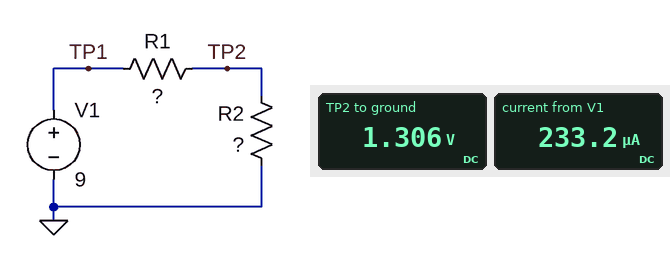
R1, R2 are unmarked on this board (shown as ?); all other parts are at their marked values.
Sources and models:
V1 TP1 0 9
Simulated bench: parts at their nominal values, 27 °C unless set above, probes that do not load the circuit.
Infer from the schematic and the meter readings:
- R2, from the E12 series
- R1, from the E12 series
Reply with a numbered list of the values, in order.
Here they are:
1. 5.6 kΩ
2. 33 kΩ
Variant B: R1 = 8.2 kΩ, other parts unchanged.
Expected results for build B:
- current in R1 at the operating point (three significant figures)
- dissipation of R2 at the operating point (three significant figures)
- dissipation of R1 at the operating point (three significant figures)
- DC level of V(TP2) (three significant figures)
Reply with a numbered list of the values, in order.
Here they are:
1. 652 µA
2. 2.38 mW
3. 3.49 mW
4. 3.65 V
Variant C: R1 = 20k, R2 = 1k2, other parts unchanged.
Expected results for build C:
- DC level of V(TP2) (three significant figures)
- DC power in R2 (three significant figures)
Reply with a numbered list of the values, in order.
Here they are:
1. 509 mV
2. 216 µW
